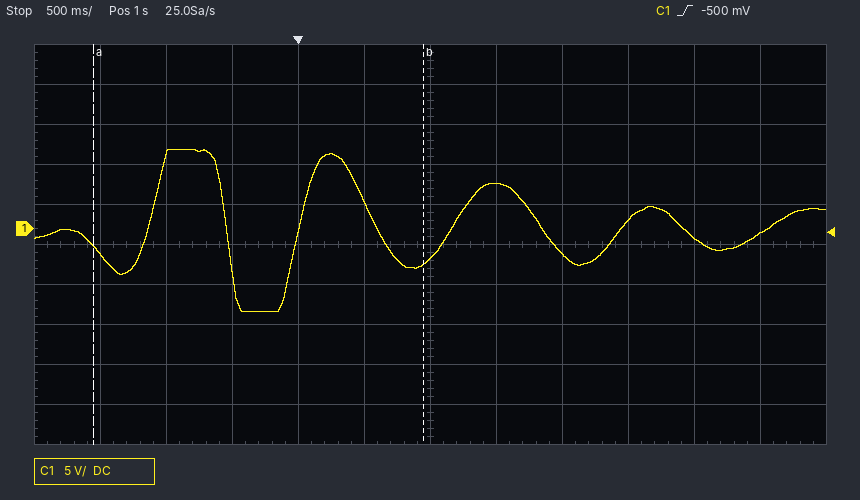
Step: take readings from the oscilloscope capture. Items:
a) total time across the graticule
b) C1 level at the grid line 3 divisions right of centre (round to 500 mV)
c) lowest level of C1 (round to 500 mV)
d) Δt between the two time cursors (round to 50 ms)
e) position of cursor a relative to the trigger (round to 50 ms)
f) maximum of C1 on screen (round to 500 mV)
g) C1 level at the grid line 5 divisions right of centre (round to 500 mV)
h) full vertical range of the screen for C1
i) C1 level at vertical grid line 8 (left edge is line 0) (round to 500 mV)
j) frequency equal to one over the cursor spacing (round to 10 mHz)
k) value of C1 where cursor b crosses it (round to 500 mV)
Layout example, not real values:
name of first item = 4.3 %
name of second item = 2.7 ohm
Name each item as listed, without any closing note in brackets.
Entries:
total time across the graticule = 6 s
C1 level at the grid line 3 divisions right of centre = 1.0 V
lowest level of C1 = -10.5 V
Δt between the two time cursors = 2.50 s
position of cursor a relative to the trigger = -1.55 s
maximum of C1 on screen = 10.0 V
C1 level at the grid line 5 divisions right of centre = -500 mV
full vertical range of the screen for C1 = 50 V
C1 level at vertical grid line 8 (left edge is line 0) = -3.0 V
frequency equal to one over the cursor spacing = 400 mHz
value of C1 where cursor b crosses it = -4.5 V
